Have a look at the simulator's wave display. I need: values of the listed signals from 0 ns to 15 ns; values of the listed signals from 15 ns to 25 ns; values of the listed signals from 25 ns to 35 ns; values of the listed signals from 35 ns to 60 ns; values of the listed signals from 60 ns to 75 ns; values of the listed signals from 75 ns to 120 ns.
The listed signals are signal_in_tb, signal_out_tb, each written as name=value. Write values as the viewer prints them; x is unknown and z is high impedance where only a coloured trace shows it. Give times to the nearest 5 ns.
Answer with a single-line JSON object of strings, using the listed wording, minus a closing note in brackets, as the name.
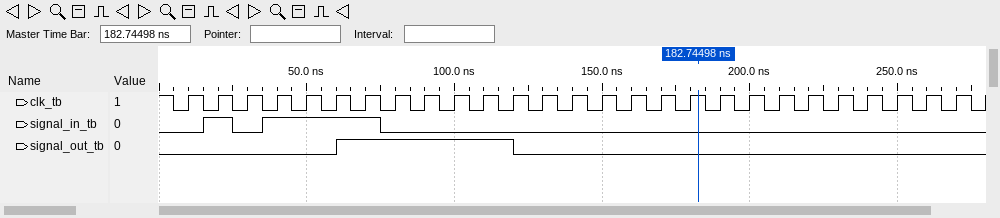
{"values of the listed signals from 0 ns to 15 ns": "signal_in_tb=0, signal_out_tb=0", "values of the listed signals from 15 ns to 25 ns": "signal_in_tb=1, signal_out_tb=0", "values of the listed signals from 25 ns to 35 ns": "signal_in_tb=0, signal_out_tb=0", "values of the listed signals from 35 ns to 60 ns": "signal_in_tb=1, signal_out_tb=0", "values of the listed signals from 60 ns to 75 ns": "signal_in_tb=1, signal_out_tb=1", "values of the listed signals from 75 ns to 120 ns": "signal_in_tb=0, signal_out_tb=1"}
